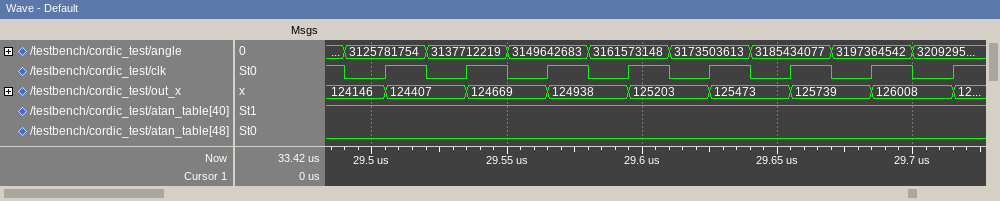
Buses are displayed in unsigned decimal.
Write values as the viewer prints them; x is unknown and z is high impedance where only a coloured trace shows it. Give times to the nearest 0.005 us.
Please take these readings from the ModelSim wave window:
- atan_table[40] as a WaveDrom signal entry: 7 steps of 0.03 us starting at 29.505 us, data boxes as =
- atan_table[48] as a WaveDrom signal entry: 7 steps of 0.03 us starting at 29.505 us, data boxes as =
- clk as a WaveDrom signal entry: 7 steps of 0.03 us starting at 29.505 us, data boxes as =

{name: 'atan_table[40]', wave: '1......'}
{name: 'atan_table[48]', wave: '0......'}
{name: 'clk', wave: 'p......'}
